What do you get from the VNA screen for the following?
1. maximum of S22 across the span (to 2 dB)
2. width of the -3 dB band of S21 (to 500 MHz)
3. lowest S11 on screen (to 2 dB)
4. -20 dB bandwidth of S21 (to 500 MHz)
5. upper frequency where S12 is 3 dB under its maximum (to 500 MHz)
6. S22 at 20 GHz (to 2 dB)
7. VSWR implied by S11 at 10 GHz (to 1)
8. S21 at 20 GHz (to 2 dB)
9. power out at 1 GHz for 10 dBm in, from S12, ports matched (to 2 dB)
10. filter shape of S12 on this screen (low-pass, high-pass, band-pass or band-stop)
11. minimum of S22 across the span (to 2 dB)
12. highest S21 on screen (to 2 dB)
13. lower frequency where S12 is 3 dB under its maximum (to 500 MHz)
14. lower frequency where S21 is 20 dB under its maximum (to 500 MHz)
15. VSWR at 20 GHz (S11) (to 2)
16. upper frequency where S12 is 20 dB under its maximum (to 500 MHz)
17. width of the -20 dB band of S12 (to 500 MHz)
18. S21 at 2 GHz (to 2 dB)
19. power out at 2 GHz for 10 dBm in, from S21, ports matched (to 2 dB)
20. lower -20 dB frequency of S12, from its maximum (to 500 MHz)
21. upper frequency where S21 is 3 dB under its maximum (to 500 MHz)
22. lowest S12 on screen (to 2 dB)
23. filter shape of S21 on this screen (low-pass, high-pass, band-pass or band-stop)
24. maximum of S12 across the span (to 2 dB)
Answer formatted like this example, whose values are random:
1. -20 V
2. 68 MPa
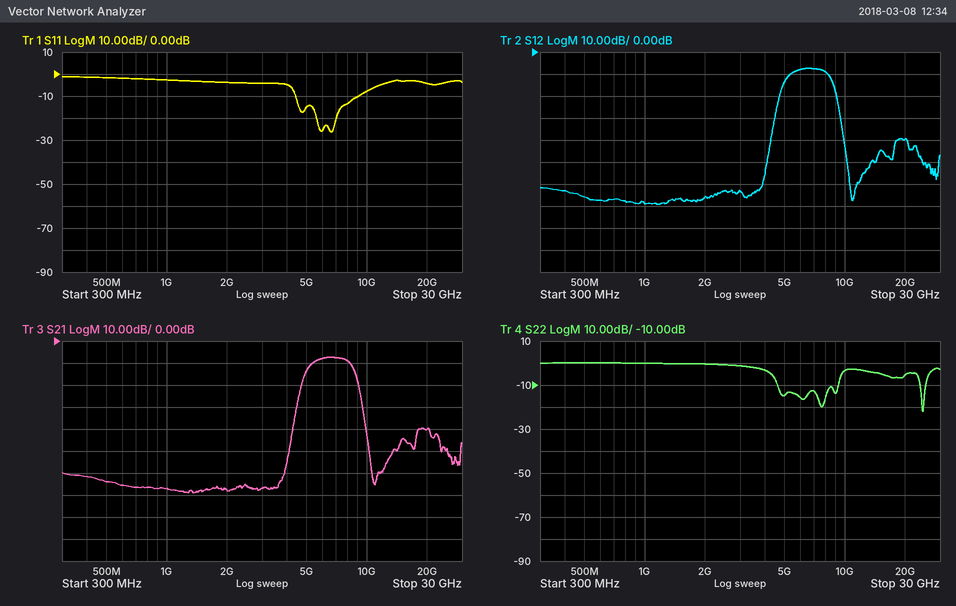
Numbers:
1. 0 dB
2. 3.0 GHz
3. -26 dB
4. 5.0 GHz
5. 8.5 GHz
6. -6 dB
7. 2
8. -40 dB
9. -58 dBm
10. band-pass
11. -22 dB
12. -8 dB
13. 5.5 GHz
14. 4.5 GHz
15. 4
16. 9.5 GHz
17. 5.0 GHz
18. -68 dB
19. -58 dBm
20. 4.5 GHz
21. 8.5 GHz
22. -70 dB
23. band-pass
24. -8 dB
